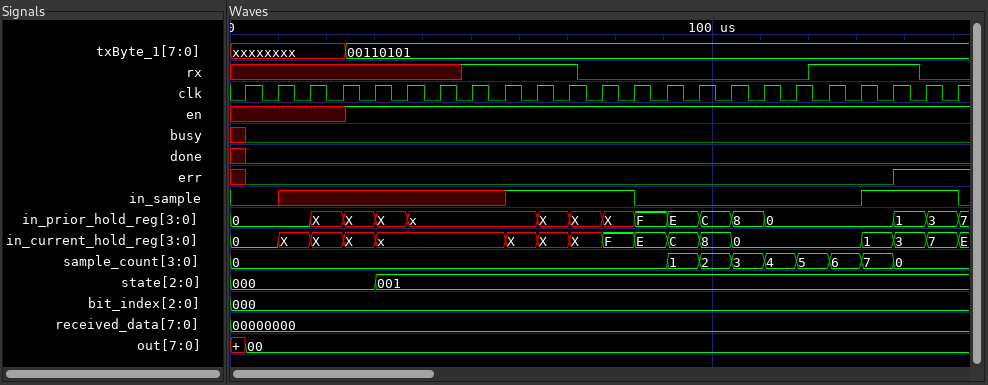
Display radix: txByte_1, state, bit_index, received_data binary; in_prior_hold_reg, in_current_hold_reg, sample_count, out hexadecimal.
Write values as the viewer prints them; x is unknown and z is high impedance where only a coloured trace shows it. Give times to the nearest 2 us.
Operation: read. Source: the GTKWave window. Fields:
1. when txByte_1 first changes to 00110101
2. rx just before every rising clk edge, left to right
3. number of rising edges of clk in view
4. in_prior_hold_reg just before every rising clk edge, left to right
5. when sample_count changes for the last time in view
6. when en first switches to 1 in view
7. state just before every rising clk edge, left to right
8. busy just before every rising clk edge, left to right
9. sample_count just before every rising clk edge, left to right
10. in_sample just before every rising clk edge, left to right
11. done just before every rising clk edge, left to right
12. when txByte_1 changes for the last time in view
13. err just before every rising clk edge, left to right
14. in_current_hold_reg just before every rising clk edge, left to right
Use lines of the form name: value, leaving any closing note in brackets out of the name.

when txByte_1 first changes to 00110101: 24 us
rx just before every rising clk edge, left to right: x x x x x x x 1 1 1 1 0 0 0 0 0 0 0 1 1 1 0 0
number of rising edges of clk in view: 23
in_prior_hold_reg just before every rising clk edge, left to right: 0, 0, 0, X, X, X, x, x, x, x, X, X, X, F, E, C, 8, 0, 0, 0, 0, 1, 3
when sample_count changes for the last time in view: 138 us
when en first switches to 1 in view: 24 us
state just before every rising clk edge, left to right: 000, 000, 000, 000, 000, 001, 001, 001, 001, 001, 001, 001, 001, 001, 001, 001, 001, 001, 001, 001, 001, 001, 001
busy just before every rising clk edge, left to right: x 0 0 0 0 0 0 0 0 0 0 0 0 0 0 0 0 0 0 0 0 0 0
sample_count just before every rising clk edge, left to right: 0, 0, 0, 0, 0, 0, 0, 0, 0, 0, 0, 0, 0, 0, 1, 2, 3, 4, 5, 6, 7, 0, 0
in_sample just before every rising clk edge, left to right: 0 0 x x x x x x x 1 1 1 1 0 0 0 0 0 0 0 1 1 1
done just before every rising clk edge, left to right: x 0 0 0 0 0 0 0 0 0 0 0 0 0 0 0 0 0 0 0 0 0 0
when txByte_1 changes for the last time in view: 24 us
err just before every rising clk edge, left to right: x 0 0 0 0 0 0 0 0 0 0 0 0 0 0 0 0 0 0 0 0 1 1
in_current_hold_reg just before every rising clk edge, left to right: 0, 0, X, X, X, x, x, x, x, X, X, X, F, E, C, 8, 0, 0, 0, 0, 1, 3, 7
